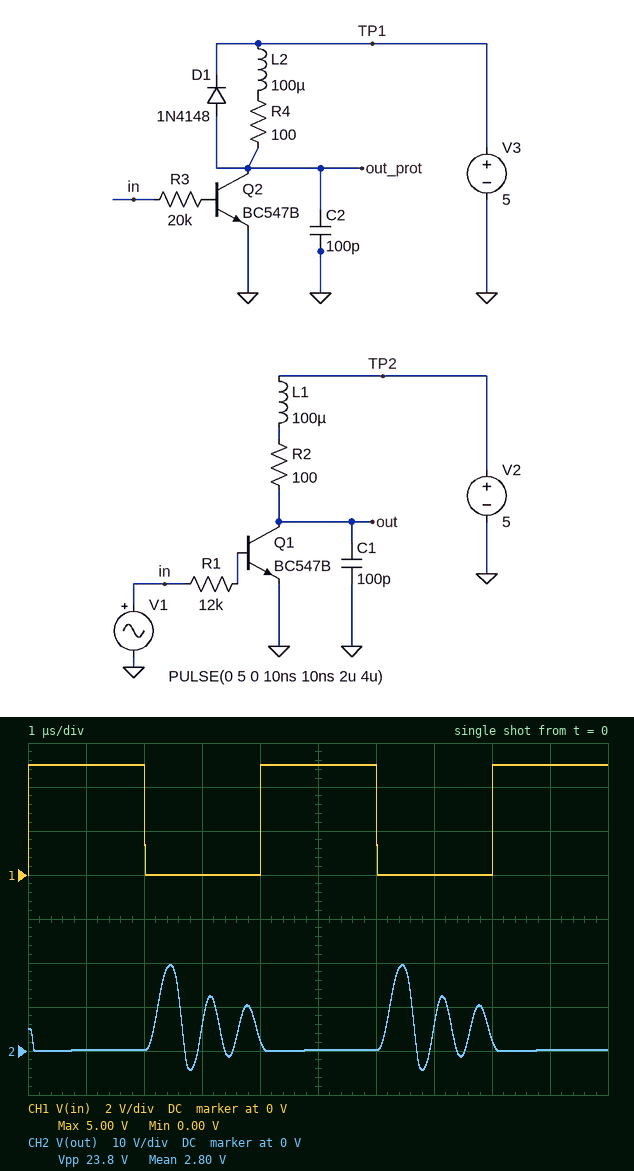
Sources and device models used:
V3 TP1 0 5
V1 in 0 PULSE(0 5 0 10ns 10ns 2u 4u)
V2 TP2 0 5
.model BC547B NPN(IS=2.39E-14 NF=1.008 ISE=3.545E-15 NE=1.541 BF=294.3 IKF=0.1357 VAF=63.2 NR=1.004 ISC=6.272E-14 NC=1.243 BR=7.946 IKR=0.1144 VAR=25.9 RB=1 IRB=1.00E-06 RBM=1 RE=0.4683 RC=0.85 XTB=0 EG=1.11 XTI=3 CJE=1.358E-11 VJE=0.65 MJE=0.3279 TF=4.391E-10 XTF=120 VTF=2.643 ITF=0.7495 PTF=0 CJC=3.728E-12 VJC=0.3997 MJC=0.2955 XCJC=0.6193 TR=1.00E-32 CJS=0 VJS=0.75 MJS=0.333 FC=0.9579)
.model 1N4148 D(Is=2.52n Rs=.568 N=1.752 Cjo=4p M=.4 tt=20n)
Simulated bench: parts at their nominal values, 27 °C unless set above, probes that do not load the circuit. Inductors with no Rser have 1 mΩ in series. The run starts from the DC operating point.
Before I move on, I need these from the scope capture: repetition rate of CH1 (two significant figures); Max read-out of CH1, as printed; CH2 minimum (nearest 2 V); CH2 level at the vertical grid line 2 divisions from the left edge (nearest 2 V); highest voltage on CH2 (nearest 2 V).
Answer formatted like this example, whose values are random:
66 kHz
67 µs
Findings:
250 kHz
5.00 V
-4 V
0 V
20 V
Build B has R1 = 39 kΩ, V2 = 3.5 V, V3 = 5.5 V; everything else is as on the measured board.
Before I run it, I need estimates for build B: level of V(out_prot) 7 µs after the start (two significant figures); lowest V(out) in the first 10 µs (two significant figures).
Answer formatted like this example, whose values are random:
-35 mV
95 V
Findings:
6.2 V
-1.3 V
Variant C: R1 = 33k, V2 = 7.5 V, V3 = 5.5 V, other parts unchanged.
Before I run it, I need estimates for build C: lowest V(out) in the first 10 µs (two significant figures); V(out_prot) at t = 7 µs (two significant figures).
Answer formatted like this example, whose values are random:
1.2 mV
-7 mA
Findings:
150 mV
6.2 V
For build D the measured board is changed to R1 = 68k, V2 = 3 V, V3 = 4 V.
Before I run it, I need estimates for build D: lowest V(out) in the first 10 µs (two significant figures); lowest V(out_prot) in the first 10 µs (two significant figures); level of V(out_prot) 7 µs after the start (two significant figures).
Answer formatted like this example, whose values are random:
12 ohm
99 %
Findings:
130 mV
39 mV
4.7 V
